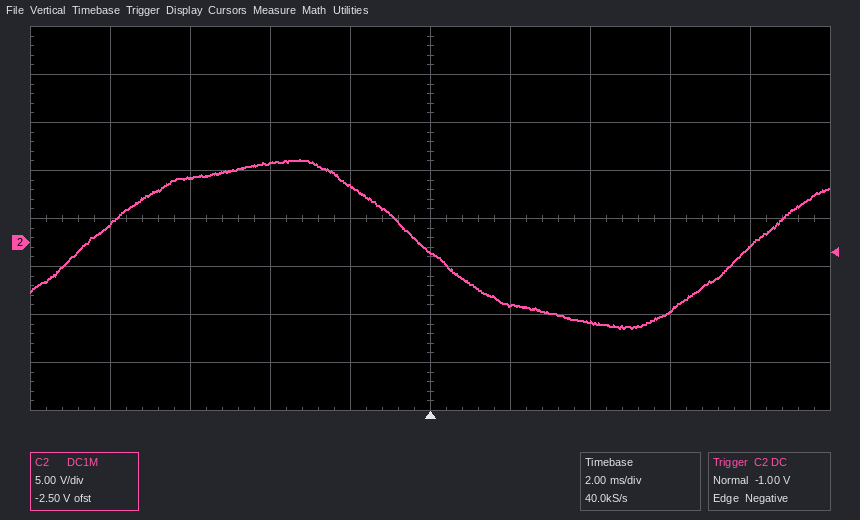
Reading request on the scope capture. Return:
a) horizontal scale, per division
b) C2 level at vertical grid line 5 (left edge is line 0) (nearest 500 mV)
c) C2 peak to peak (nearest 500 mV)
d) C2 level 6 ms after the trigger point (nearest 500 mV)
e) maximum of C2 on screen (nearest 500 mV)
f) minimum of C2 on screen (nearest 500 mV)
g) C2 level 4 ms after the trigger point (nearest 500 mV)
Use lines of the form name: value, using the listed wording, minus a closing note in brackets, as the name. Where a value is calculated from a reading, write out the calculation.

horizontal scale, per division: 2 ms
C2 level at vertical grid line 5 (left edge is line 0): -1.0 V
C2 peak to peak: 8.5 V − (-9.0 V) = 17.5 V
C2 level 6 ms after the trigger point: -7.0 V
maximum of C2 on screen: 8.5 V
minimum of C2 on screen: -9.0 V
C2 level 4 ms after the trigger point: -8.5 V
